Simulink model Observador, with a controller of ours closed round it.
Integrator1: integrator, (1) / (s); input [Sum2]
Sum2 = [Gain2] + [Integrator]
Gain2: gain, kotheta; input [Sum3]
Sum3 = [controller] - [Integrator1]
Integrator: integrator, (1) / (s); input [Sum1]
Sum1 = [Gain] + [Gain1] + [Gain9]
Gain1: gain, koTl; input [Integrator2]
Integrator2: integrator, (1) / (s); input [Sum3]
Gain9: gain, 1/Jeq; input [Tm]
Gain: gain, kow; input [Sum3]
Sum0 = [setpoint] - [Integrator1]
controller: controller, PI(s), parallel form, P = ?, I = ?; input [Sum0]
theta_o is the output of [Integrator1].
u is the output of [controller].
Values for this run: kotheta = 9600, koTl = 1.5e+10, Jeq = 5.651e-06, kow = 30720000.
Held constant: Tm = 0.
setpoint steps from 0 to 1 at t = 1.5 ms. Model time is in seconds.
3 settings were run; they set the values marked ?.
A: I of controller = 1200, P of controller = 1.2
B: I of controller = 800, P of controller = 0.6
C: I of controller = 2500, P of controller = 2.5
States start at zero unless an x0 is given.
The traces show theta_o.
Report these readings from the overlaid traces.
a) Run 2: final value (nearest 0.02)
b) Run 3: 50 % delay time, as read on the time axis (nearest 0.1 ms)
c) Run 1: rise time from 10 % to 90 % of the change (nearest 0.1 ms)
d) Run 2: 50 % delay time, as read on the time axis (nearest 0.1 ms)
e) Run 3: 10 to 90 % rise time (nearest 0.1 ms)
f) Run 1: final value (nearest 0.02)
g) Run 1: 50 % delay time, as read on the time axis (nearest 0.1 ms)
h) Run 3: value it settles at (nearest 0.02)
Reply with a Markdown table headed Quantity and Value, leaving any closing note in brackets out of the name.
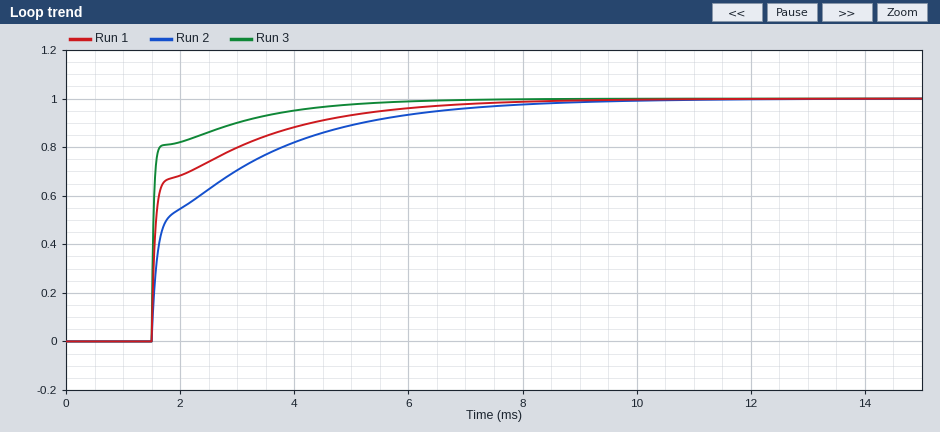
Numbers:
| Quantity | Value |
|---|---|
| Run 2: final value | 1.00 |
| Run 3: 50 % delay time, as read on the time axis | 1.5 ms |
| Run 1: rise time from 10 % to 90 % of the change | 2.8 ms |
| Run 2: 50 % delay time, as read on the time axis | 1.8 ms |
| Run 3: 10 to 90 % rise time | 1.5 ms |
| Run 1: final value | 1.00 |
| Run 1: 50 % delay time, as read on the time axis | 1.6 ms |
| Run 3: value it settles at | 1.00 |
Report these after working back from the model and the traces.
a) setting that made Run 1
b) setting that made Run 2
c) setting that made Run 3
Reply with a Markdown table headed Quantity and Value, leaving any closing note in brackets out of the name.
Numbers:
| Quantity | Value |
|---|---|
| setting that made Run 1 | A |
| setting that made Run 2 | B |
| setting that made Run 3 | C |
